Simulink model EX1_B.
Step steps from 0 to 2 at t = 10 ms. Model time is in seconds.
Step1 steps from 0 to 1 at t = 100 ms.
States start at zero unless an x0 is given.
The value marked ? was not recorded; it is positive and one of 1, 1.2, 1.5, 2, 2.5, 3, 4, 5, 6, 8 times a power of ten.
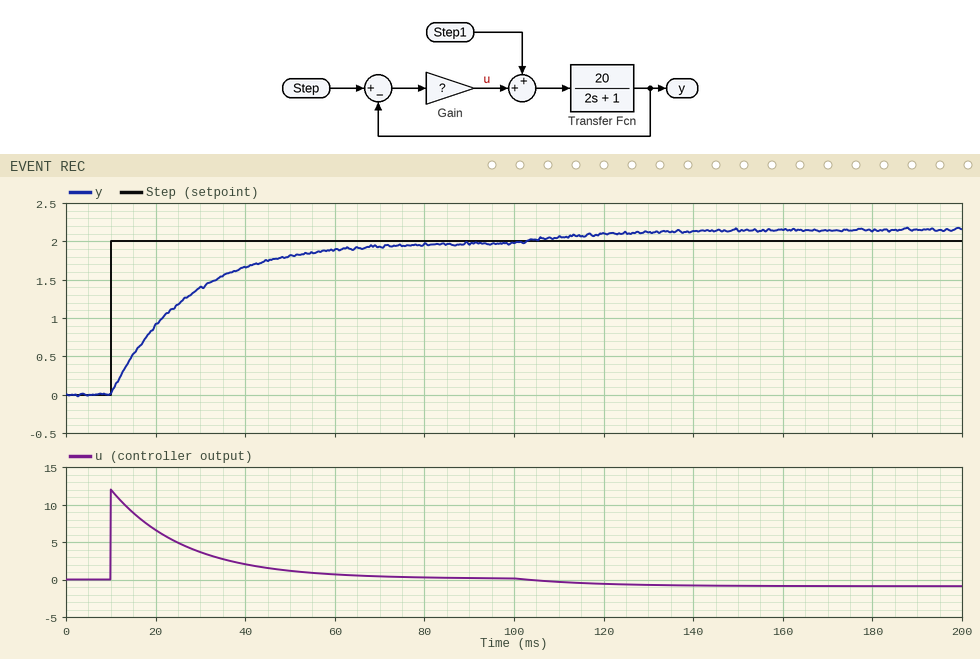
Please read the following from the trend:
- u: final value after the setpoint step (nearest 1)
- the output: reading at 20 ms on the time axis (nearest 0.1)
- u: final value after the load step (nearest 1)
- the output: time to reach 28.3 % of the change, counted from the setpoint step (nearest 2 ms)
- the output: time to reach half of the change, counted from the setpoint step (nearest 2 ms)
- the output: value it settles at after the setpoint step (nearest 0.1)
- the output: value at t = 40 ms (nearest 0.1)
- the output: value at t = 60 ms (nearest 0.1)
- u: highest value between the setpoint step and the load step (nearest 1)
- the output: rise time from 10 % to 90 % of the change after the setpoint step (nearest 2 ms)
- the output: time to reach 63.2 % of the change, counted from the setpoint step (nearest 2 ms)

0
0.9
-1
6 ms
12 ms
2.0
1.7
1.9
12
36 ms
16 ms
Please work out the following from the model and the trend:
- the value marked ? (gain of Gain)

6
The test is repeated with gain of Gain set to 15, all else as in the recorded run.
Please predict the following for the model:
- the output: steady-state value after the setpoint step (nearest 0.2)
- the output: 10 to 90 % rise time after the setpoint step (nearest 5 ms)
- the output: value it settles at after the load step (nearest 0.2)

2.0
15 ms
2.0
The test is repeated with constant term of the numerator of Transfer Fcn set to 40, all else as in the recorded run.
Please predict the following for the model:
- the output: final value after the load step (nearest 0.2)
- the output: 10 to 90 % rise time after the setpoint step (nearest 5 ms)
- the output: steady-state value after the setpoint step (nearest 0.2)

2.2
20 ms
2.0
